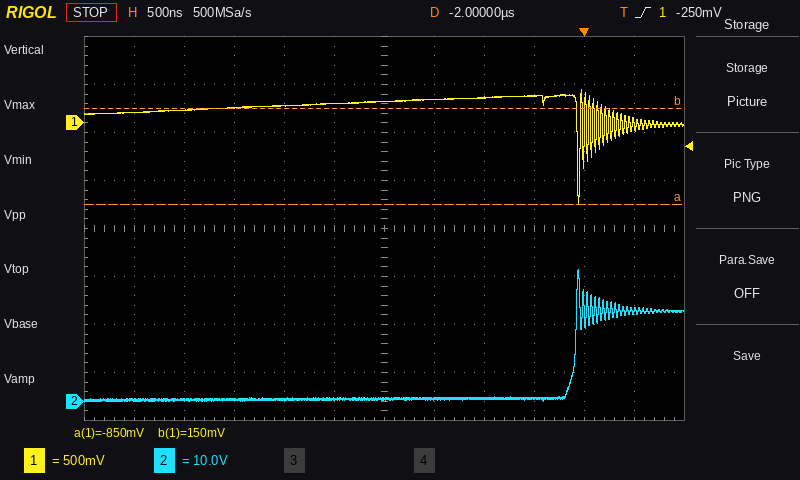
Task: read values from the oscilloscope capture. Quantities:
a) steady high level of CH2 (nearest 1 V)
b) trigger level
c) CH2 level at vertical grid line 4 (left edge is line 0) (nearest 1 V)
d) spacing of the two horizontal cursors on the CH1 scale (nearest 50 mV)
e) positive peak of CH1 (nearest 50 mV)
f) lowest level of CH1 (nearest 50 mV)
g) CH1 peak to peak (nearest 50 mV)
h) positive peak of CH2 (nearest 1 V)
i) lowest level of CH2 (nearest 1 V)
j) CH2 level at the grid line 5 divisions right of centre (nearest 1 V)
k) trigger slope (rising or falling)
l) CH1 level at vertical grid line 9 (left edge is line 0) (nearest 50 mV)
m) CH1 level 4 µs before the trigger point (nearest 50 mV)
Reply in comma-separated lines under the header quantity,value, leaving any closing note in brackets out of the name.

quantity,value
steady high level of CH2,19 V
trigger level,-250 mV
CH2 level at vertical grid line 4 (left edge is line 0),0 V
spacing of the two horizontal cursors on the CH1 scale,1.00 V
positive peak of CH1,350 mV
lowest level of CH1,-850 mV
CH1 peak to peak,1.20 V
positive peak of CH2,27 V
lowest level of CH2,0 V
CH2 level at the grid line 5 divisions right of centre,19 V
trigger slope,rising
CH1 level at vertical grid line 9 (left edge is line 0),300 mV
CH1 level 4 µs before the trigger point,150 mV
